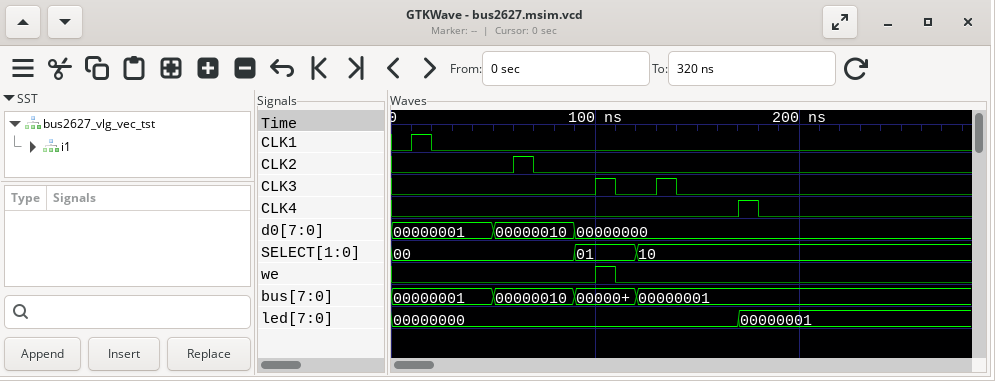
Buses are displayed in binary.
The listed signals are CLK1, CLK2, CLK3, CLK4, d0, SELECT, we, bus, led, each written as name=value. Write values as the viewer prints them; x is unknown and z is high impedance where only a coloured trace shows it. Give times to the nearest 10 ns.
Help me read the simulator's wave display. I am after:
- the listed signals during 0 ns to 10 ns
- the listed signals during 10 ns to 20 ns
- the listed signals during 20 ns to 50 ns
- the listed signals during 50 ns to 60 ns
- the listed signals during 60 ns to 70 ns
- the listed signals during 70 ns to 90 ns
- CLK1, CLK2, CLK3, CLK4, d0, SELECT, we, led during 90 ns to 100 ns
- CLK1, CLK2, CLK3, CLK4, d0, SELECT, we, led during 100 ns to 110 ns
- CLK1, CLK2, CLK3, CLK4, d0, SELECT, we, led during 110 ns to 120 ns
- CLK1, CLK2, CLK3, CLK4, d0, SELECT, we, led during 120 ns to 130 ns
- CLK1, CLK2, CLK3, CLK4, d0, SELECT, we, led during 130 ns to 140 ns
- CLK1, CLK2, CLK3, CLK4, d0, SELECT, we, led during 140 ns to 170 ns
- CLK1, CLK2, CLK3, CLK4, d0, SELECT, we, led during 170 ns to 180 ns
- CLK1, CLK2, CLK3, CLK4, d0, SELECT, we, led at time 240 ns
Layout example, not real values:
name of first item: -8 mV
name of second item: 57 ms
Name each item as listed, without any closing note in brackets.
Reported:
the listed signals during 0 ns to 10 ns: CLK1=0, CLK2=0, CLK3=0, CLK4=0, d0=00000001, SELECT=00, we=0, bus=00000001, led=00000000
the listed signals during 10 ns to 20 ns: CLK1=1, CLK2=0, CLK3=0, CLK4=0, d0=00000001, SELECT=00, we=0, bus=00000001, led=00000000
the listed signals during 20 ns to 50 ns: CLK1=0, CLK2=0, CLK3=0, CLK4=0, d0=00000001, SELECT=00, we=0, bus=00000001, led=00000000
the listed signals during 50 ns to 60 ns: CLK1=0, CLK2=0, CLK3=0, CLK4=0, d0=00000010, SELECT=00, we=0, bus=00000010, led=00000000
the listed signals during 60 ns to 70 ns: CLK1=0, CLK2=1, CLK3=0, CLK4=0, d0=00000010, SELECT=00, we=0, bus=00000010, led=00000000
the listed signals during 70 ns to 90 ns: CLK1=0, CLK2=0, CLK3=0, CLK4=0, d0=00000010, SELECT=00, we=0, bus=00000010, led=00000000
CLK1, CLK2, CLK3, CLK4, d0, SELECT, we, led during 90 ns to 100 ns: CLK1=0, CLK2=0, CLK3=0, CLK4=0, d0=00000000, SELECT=01, we=0, led=00000000
CLK1, CLK2, CLK3, CLK4, d0, SELECT, we, led during 100 ns to 110 ns: CLK1=0, CLK2=0, CLK3=1, CLK4=0, d0=00000000, SELECT=01, we=1, led=00000000
CLK1, CLK2, CLK3, CLK4, d0, SELECT, we, led during 110 ns to 120 ns: CLK1=0, CLK2=0, CLK3=0, CLK4=0, d0=00000000, SELECT=01, we=0, led=00000000
CLK1, CLK2, CLK3, CLK4, d0, SELECT, we, led during 120 ns to 130 ns: CLK1=0, CLK2=0, CLK3=0, CLK4=0, d0=00000000, SELECT=10, we=0, led=00000000
CLK1, CLK2, CLK3, CLK4, d0, SELECT, we, led during 130 ns to 140 ns: CLK1=0, CLK2=0, CLK3=1, CLK4=0, d0=00000000, SELECT=10, we=0, led=00000000
CLK1, CLK2, CLK3, CLK4, d0, SELECT, we, led during 140 ns to 170 ns: CLK1=0, CLK2=0, CLK3=0, CLK4=0, d0=00000000, SELECT=10, we=0, led=00000000
CLK1, CLK2, CLK3, CLK4, d0, SELECT, we, led during 170 ns to 180 ns: CLK1=0, CLK2=0, CLK3=0, CLK4=1, d0=00000000, SELECT=10, we=0, led=00000001
CLK1, CLK2, CLK3, CLK4, d0, SELECT, we, led at time 240 ns: CLK1=0, CLK2=0, CLK3=0, CLK4=0, d0=00000000, SELECT=10, we=0, led=00000001
